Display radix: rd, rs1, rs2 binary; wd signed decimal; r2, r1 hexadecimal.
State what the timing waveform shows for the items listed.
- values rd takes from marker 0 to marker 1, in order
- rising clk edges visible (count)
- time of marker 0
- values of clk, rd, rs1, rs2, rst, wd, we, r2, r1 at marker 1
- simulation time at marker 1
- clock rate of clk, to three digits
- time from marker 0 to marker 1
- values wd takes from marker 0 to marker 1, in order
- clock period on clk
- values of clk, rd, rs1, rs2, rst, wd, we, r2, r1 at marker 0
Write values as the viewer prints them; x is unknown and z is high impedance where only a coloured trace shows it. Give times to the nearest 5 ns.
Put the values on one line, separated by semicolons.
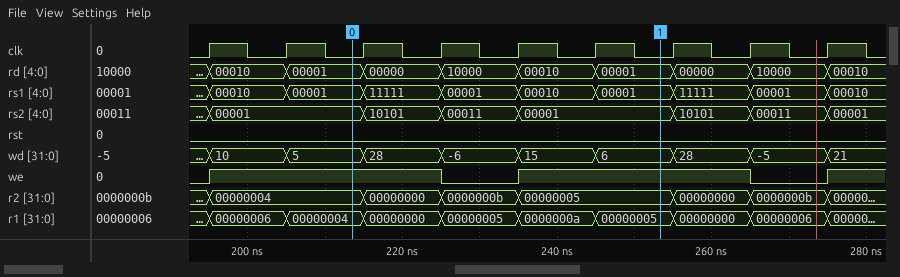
00001, 00000, 10000, 00010, 00001; 9; 215 ns; clk=0, rd=00001, rs1=00001, rs2=00001, rst=0, wd=6, we=1, r2=00000005, r1=00000005; 255 ns; 100 MHz; 40 ns; 5, 28, -6, 15, 6; 10 ns; clk=0, rd=00001, rs1=00001, rs2=00001, rst=0, wd=5, we=1, r2=00000004, r1=00000004
